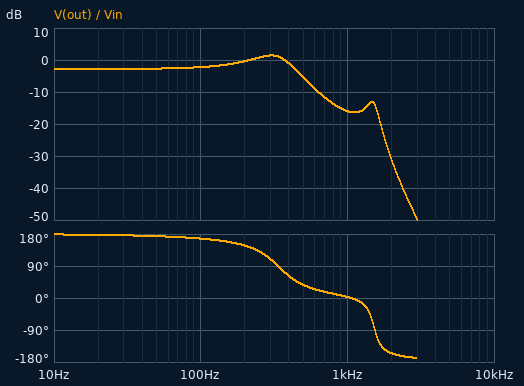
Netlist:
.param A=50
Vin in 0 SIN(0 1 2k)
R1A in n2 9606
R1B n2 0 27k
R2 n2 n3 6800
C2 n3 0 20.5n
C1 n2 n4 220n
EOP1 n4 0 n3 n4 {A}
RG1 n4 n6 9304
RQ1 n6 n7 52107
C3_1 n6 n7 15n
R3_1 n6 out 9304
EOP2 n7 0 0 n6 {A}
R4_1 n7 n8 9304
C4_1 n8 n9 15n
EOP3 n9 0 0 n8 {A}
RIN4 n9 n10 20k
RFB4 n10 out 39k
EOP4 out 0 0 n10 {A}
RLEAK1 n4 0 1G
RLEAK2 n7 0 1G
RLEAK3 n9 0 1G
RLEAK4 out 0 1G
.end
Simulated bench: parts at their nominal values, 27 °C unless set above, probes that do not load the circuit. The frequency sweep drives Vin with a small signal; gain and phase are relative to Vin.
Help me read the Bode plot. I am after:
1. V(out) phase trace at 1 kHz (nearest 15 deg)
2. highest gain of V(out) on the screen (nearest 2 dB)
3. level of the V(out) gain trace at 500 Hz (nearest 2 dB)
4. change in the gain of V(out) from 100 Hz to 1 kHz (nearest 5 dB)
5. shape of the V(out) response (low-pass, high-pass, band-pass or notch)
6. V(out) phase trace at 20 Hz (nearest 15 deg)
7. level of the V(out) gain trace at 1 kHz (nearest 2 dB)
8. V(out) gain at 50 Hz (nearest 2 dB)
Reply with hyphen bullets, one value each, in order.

- 0 deg
- 2 dB
- -6 dB
- -15 dB
- low-pass
- 180 deg
- -16 dB
- -2 dB
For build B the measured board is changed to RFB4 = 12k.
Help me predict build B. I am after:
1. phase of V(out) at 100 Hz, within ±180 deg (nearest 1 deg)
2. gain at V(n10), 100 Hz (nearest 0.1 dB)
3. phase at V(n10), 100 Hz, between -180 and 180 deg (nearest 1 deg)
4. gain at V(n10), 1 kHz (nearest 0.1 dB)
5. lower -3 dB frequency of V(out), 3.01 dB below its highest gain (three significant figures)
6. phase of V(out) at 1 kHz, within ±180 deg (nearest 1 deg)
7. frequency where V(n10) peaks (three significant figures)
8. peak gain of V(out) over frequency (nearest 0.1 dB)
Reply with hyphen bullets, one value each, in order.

- 166 deg
- -36.2 dB
- -14 deg
- -49.1 dB
- 171 Hz
- -120 deg
- 313 Hz
- 2.2 dB
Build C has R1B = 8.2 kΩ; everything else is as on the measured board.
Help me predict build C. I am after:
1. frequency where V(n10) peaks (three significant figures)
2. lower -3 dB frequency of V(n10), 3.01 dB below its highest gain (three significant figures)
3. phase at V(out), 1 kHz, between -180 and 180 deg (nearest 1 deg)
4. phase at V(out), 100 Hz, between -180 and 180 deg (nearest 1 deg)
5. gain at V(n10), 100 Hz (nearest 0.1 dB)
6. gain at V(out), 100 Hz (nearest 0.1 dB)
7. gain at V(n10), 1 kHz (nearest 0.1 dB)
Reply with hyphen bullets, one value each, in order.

- 388 Hz
- 192 Hz
- 8 deg
- 170 deg
- -40.5 dB
- -6.5 dB
- -49.5 dB
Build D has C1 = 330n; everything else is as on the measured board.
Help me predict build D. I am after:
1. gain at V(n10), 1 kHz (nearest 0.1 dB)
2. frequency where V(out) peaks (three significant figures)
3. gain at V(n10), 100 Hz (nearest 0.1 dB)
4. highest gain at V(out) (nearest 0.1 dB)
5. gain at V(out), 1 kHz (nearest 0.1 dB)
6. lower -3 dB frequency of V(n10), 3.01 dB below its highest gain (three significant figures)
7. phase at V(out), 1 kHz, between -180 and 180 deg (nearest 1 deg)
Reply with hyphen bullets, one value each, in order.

- -53.7 dB
- 256 Hz
- -35.8 dB
- 2.5 dB
- -19.7 dB
- 152 Hz
- -2 deg
